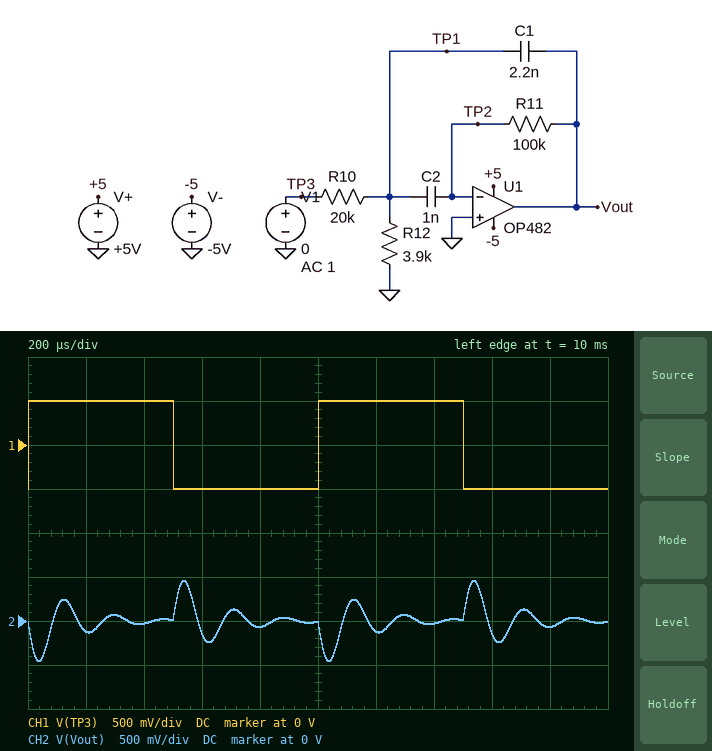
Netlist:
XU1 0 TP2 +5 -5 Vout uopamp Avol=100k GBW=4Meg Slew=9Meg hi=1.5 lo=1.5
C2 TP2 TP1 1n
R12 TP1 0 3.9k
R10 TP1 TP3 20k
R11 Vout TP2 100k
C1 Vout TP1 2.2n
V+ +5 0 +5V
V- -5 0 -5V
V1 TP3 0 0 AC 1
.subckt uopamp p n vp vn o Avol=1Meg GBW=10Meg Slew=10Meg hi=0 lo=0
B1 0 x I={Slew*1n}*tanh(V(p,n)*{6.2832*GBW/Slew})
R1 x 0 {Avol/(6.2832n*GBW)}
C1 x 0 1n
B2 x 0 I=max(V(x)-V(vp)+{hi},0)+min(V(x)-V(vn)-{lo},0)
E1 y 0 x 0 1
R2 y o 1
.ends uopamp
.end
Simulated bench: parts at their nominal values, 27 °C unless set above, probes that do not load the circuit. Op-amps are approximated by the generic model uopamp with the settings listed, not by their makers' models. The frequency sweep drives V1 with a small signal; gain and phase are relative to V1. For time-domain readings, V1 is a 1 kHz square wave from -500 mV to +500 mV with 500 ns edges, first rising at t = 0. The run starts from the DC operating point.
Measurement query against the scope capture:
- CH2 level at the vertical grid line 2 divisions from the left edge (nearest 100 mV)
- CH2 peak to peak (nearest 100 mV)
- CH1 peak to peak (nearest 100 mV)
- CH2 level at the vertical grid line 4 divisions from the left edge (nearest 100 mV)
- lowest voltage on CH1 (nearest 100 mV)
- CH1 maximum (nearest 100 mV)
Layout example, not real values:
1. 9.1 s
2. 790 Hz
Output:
1. 0 V
2. 900 mV
3. 1.0 V
4. -100 mV
5. -500 mV
6. 500 mV
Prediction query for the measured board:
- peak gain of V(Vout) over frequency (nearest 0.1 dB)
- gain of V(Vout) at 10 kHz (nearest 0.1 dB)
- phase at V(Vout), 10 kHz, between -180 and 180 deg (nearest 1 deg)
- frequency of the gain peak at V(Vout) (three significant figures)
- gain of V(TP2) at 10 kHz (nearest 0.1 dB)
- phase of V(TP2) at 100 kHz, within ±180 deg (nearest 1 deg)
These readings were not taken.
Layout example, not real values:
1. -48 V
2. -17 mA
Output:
1. 3.9 dB
2. -5.6 dB
3. 109 deg
4. 5.92 kHz
5. -57.7 dB
6. 0 deg
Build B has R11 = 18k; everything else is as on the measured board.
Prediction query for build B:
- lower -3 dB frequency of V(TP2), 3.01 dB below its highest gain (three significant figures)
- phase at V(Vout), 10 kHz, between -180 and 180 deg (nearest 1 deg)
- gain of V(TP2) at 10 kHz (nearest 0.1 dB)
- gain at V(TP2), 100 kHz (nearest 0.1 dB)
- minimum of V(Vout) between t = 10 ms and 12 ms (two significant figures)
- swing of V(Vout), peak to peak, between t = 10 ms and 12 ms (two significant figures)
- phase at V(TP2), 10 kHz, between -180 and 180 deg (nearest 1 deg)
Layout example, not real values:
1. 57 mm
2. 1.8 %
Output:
1. 11.8 kHz
2. -144 deg
3. -65.0 dB
4. -60.8 dB
5. -150 mV
6. 290 mV
7. 126 deg
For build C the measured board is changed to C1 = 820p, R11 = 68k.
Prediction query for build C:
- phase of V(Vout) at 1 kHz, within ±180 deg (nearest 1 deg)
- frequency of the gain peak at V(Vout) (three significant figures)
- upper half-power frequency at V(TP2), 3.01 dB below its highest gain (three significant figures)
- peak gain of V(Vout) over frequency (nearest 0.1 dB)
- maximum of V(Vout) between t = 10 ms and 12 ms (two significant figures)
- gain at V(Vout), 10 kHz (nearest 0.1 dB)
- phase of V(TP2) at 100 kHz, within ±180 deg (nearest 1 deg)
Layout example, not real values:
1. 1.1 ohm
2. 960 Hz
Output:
1. -92 deg
2. 11.7 kHz
3. 16.9 kHz
4. 5.4 dB
5. 600 mV
6. 3.6 dB
7. 2 deg
